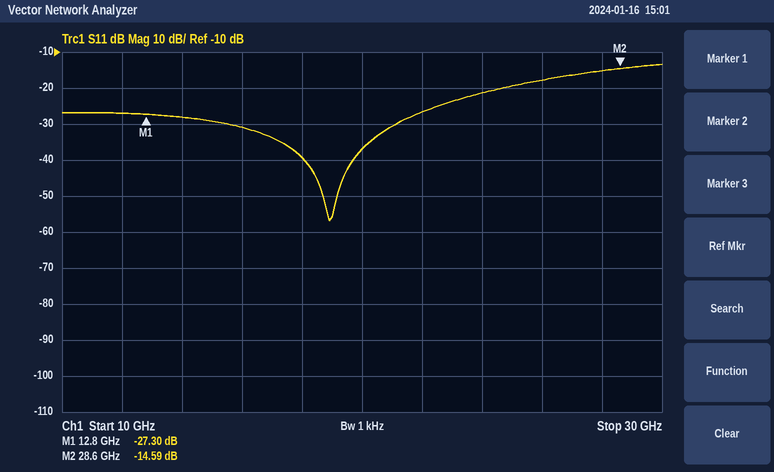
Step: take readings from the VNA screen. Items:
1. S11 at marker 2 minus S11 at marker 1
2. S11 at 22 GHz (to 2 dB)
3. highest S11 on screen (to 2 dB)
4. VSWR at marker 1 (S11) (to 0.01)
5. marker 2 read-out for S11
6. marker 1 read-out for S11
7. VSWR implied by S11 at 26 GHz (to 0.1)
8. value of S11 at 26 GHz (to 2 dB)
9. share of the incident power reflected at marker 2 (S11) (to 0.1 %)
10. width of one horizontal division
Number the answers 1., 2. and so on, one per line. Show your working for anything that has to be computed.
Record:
1. -14.59 − (-27.3) = 12.71 dB
2. -26 dB
3. -14 dB
4. (1 + 0.0432)/(1 − 0.0432) ≈ 1.09
5. -14.59 dB
6. -27.30 dB
7. |Γ| = 10^(-18/20) = 0.1259; VSWR = (1 + 0.1259)/(1 − 0.1259) ≈ 1.3
8. -18 dB
9. 10^(-14.59/10) ≈ 3.5 %
10. 2 GHz
